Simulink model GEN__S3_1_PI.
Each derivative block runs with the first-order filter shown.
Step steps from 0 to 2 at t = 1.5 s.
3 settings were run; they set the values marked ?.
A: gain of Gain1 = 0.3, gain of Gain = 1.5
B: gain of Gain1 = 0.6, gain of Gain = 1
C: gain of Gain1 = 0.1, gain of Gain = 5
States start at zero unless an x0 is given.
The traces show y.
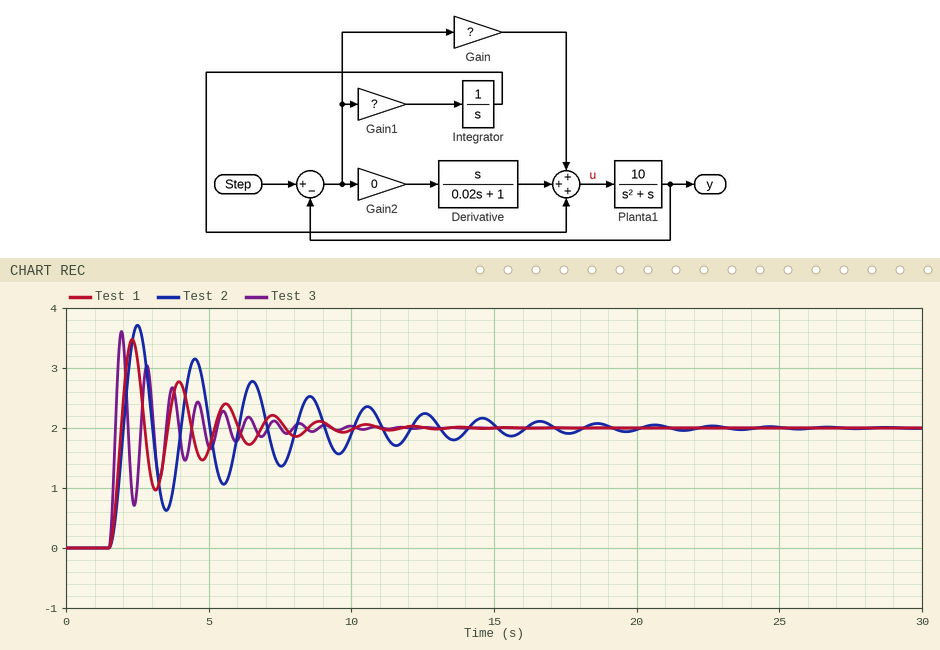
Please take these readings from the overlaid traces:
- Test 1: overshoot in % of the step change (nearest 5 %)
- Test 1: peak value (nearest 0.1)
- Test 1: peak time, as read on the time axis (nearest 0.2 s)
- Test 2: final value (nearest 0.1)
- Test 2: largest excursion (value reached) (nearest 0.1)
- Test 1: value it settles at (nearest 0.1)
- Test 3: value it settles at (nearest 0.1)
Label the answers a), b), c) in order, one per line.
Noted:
a) 75 %
b) 3.5
c) 2.4 s
d) 2.0
e) 3.7
f) 2.0
g) 2.0
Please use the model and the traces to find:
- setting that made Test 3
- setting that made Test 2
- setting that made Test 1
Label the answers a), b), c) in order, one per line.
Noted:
a) C
b) B
c) A
